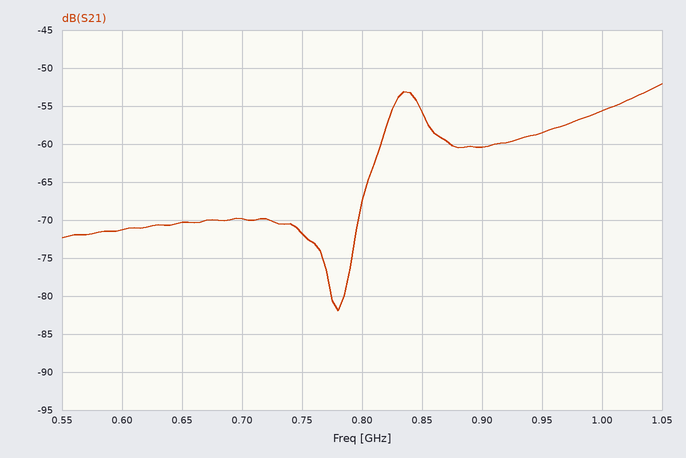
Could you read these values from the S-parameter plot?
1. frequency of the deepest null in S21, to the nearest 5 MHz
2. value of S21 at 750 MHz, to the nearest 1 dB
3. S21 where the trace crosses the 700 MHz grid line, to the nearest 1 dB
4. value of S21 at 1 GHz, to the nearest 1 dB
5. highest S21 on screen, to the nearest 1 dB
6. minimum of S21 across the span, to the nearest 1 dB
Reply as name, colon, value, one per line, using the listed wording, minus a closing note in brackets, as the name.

frequency of the deepest null in S21, to the nearest 5 MHz: 780 MHz
value of S21 at 750 MHz, to the nearest 1 dB: -72 dB
S21 where the trace crosses the 700 MHz grid line, to the nearest 1 dB: -70 dB
value of S21 at 1 GHz, to the nearest 1 dB: -56 dB
highest S21 on screen, to the nearest 1 dB: -52 dB
minimum of S21 across the span, to the nearest 1 dB: -82 dB
